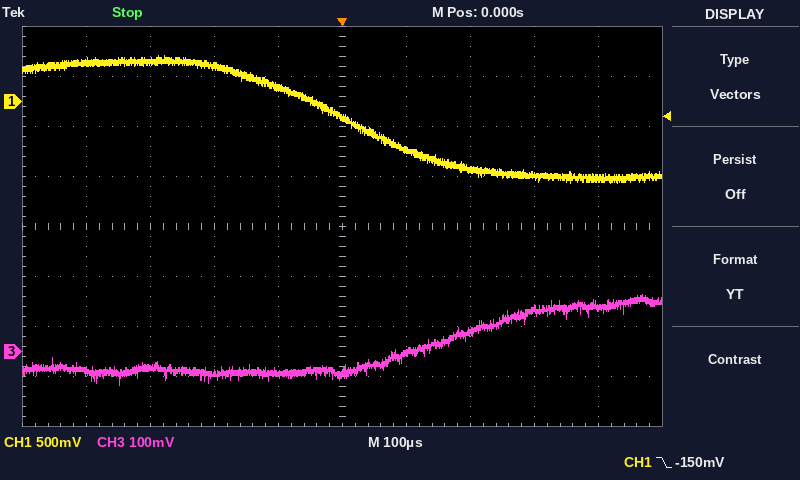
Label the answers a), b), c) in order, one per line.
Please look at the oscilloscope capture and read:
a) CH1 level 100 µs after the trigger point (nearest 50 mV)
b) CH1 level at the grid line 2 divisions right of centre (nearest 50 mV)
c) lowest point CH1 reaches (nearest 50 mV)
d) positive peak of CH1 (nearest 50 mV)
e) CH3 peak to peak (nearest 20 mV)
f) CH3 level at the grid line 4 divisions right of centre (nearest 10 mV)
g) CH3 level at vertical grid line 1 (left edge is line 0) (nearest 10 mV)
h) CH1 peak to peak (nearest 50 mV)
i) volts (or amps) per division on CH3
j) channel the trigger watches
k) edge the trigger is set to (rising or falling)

a) -500 mV
b) -700 mV
c) -800 mV
d) 450 mV
e) 180 mV
f) 90 mV
g) -40 mV
h) 1.25 V
i) 100 mV
j) CH1
k) falling
